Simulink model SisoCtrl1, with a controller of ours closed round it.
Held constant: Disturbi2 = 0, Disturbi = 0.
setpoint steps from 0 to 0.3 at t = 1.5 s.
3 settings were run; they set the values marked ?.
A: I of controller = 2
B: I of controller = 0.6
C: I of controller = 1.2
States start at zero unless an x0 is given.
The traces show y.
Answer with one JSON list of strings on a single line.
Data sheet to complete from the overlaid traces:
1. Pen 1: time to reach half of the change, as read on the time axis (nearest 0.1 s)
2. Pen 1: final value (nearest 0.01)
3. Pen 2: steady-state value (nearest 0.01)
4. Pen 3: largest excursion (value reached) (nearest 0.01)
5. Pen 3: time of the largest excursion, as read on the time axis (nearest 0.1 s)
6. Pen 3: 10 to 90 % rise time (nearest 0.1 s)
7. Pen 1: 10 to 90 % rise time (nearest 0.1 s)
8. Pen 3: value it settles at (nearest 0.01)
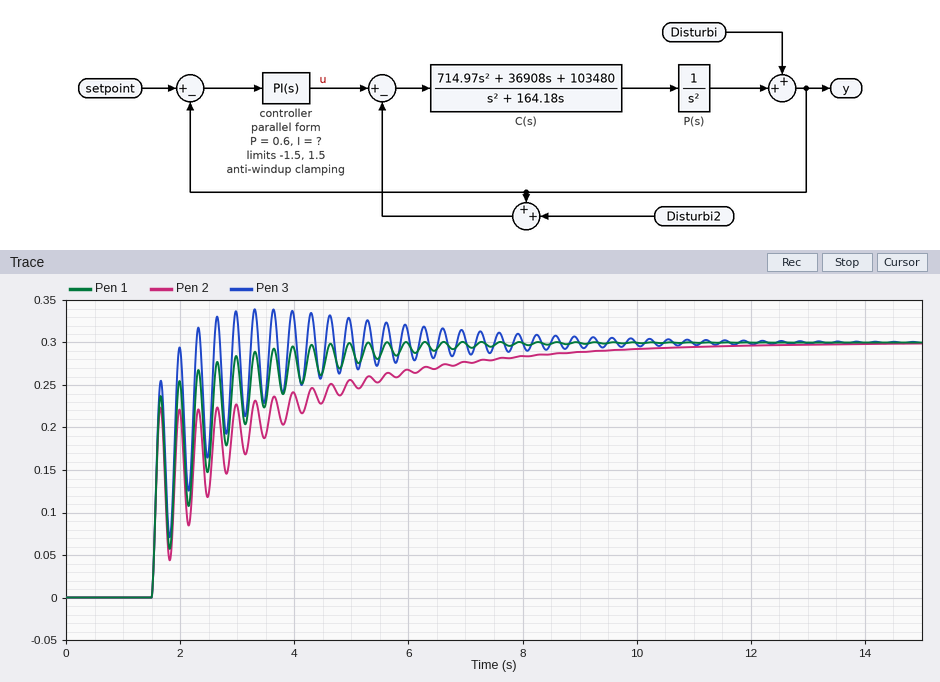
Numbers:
["1.6 s", "0.30", "0.30", "0.34", "3.3 s", "0.4 s", "1.1 s", "0.30"]
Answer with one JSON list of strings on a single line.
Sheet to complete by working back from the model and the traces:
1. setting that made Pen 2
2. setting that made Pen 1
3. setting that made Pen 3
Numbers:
["B", "C", "A"]
